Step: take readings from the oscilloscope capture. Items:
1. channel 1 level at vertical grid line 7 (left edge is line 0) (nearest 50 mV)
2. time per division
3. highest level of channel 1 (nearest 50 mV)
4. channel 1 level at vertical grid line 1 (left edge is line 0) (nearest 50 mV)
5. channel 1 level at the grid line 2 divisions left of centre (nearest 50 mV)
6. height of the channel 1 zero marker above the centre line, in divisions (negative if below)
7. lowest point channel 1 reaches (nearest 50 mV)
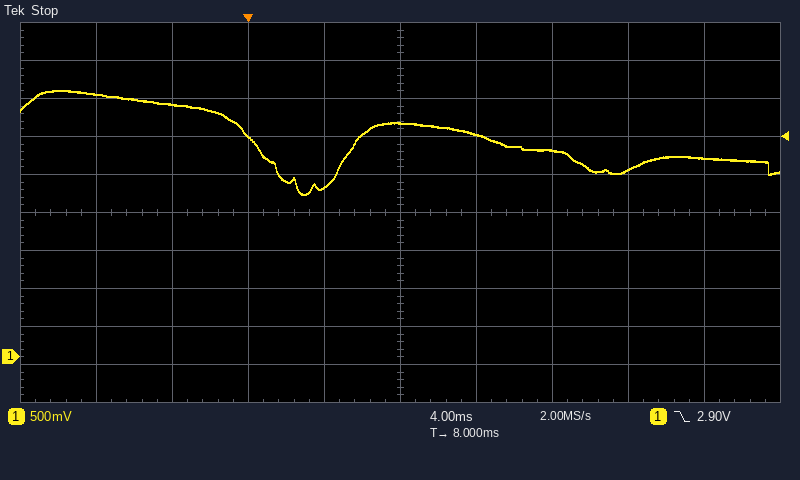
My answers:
2.70 V
4 ms
3.50 V
3.45 V
2.90 V
-3.8 div
2.15 V
